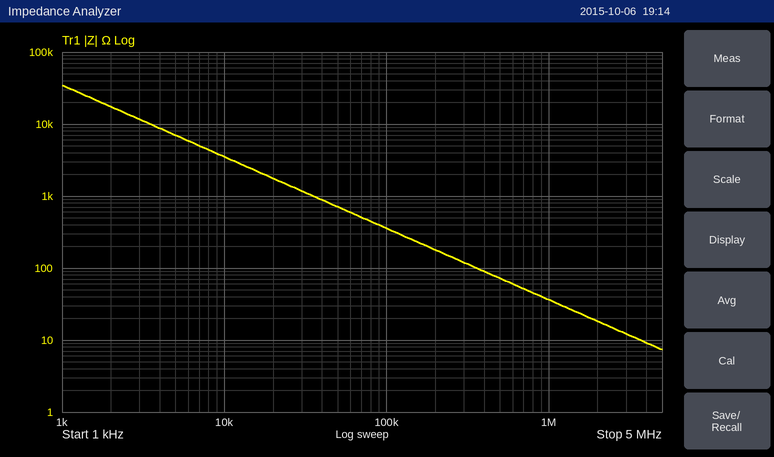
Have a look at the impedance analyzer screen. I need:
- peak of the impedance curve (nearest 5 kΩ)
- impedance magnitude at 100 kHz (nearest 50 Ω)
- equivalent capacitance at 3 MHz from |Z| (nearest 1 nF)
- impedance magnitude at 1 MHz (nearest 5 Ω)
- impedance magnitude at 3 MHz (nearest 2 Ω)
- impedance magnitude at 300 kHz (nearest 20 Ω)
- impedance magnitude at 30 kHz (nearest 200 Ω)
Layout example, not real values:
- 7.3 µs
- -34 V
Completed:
- 35 kΩ
- 350 Ω
- 4 nF
- 35 Ω
- 12 Ω
- 120 Ω
- 1.2 kΩ
